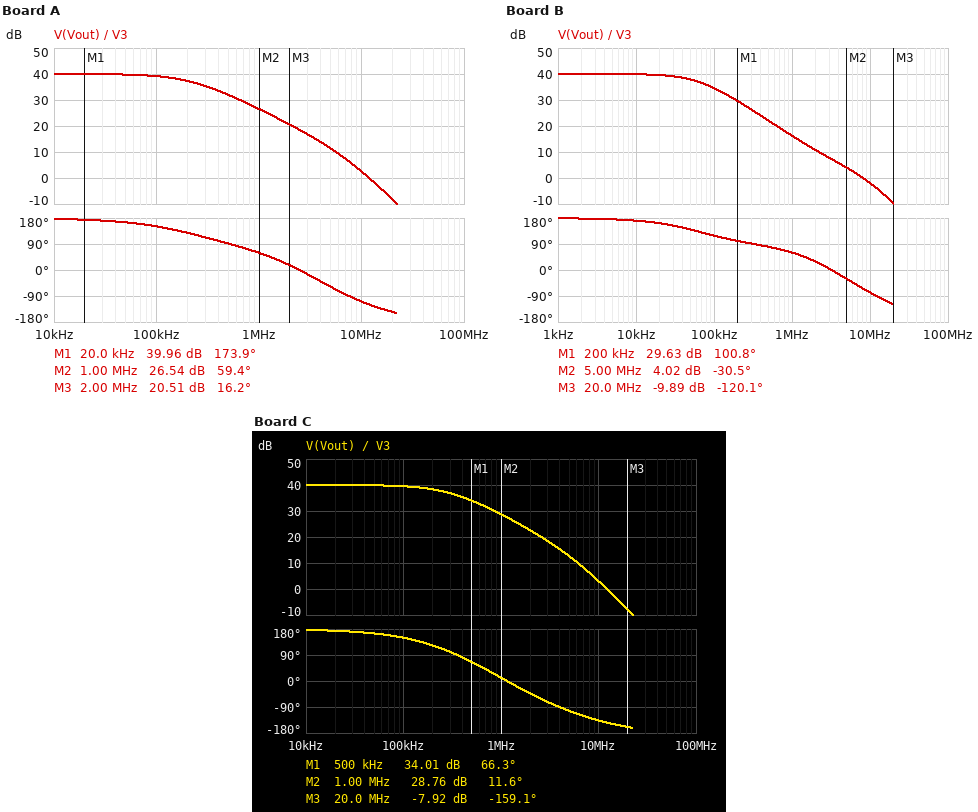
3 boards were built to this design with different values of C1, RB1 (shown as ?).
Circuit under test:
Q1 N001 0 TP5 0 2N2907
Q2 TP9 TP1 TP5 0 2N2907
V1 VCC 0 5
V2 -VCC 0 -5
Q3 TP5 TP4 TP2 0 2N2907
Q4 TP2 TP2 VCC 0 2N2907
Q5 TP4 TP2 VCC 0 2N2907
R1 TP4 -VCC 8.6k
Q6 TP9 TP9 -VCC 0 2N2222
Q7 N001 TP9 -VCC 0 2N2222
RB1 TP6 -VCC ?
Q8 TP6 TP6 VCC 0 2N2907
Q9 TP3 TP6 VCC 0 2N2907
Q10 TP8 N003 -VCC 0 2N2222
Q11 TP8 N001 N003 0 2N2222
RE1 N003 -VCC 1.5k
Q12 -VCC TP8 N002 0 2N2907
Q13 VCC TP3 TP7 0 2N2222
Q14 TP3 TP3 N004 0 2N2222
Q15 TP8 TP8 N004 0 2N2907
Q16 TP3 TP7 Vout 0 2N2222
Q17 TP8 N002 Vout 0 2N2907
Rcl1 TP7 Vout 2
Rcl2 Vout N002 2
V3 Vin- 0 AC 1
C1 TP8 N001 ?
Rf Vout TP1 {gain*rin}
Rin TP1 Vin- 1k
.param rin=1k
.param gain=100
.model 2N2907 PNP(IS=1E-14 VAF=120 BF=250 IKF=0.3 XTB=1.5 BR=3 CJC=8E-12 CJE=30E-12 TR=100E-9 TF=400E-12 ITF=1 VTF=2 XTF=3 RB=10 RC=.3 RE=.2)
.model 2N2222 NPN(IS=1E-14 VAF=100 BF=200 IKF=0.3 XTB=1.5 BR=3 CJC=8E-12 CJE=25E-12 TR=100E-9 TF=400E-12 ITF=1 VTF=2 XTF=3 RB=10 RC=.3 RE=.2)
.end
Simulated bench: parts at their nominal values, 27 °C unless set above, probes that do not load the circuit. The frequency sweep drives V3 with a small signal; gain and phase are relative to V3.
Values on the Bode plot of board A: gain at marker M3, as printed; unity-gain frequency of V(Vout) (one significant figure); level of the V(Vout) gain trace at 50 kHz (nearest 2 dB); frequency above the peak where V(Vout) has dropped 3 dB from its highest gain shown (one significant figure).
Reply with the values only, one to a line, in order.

20.51 dB
10 MHz
40 dB
200 kHz
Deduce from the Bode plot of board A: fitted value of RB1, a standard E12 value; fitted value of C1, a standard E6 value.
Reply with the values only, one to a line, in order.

22 kΩ
150 pF
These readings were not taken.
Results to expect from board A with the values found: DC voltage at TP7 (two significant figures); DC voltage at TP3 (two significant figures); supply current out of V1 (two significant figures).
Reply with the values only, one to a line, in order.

-180 mV
450 mV
3.3 mA
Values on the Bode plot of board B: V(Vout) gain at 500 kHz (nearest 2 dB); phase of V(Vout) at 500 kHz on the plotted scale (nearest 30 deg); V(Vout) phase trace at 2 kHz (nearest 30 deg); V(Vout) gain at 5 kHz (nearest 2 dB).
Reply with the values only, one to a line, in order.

22 dB
90 deg
180 deg
40 dB
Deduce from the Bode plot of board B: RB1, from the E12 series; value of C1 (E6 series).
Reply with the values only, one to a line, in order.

15 kΩ
470 pF
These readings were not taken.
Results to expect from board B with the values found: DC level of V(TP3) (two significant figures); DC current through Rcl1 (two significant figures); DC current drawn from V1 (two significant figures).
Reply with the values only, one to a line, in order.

460 mV
630 µA
3.9 mA
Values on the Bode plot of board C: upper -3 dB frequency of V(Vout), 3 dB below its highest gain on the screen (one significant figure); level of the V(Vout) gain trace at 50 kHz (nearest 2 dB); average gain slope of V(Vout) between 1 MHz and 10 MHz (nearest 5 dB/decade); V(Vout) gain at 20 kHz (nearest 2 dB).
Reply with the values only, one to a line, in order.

300 kHz
40 dB
-25 dB/decade
40 dB
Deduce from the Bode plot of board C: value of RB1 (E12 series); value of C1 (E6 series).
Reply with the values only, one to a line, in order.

27 kΩ
150 pF
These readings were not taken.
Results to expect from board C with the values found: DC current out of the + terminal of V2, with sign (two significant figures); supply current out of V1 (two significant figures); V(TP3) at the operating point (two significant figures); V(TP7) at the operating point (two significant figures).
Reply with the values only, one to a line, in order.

-3.1 mA
3.1 mA
440 mV
-190 mV
